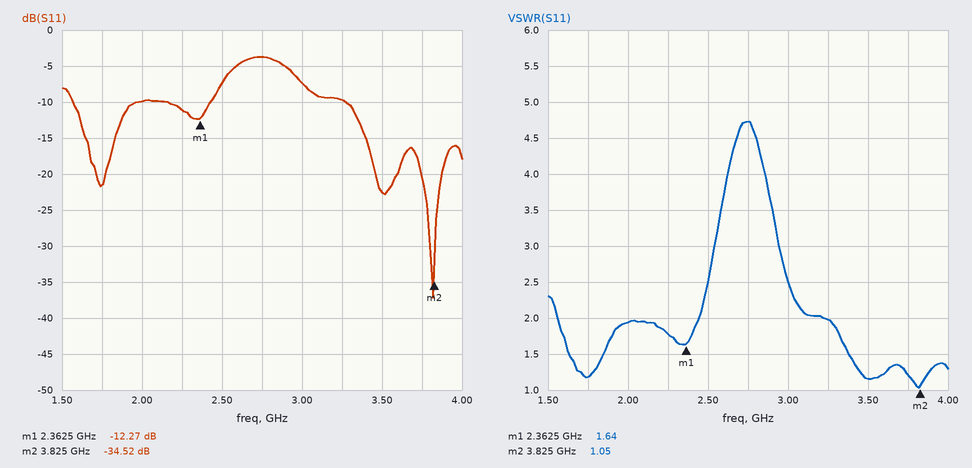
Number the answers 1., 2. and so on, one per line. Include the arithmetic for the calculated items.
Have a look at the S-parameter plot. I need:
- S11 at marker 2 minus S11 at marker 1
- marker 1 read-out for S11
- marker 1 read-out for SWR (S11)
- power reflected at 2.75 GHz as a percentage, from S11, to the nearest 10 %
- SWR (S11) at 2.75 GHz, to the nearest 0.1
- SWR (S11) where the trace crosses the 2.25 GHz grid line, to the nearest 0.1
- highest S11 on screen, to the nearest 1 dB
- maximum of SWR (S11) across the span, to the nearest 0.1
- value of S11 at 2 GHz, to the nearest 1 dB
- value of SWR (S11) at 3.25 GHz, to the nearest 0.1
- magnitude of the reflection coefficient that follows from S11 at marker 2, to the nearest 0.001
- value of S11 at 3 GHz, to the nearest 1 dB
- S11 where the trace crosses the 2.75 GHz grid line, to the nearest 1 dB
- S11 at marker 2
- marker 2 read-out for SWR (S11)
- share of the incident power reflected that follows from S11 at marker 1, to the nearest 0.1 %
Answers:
1. -34.52 − (-12.27) = -22.25 dB
2. -12.27 dB
3. 1.64
4. 10^(-4/10) ≈ 40 %
5. 4.7
6. 1.8
7. -4 dB
8. 4.7
9. -10 dB
10. 2.0
11. 10^(-34.52/20) ≈ 0.019
12. -7 dB
13. -4 dB
14. -34.52 dB
15. 1.05
16. 10^(-12.27/10) ≈ 5.9 %
